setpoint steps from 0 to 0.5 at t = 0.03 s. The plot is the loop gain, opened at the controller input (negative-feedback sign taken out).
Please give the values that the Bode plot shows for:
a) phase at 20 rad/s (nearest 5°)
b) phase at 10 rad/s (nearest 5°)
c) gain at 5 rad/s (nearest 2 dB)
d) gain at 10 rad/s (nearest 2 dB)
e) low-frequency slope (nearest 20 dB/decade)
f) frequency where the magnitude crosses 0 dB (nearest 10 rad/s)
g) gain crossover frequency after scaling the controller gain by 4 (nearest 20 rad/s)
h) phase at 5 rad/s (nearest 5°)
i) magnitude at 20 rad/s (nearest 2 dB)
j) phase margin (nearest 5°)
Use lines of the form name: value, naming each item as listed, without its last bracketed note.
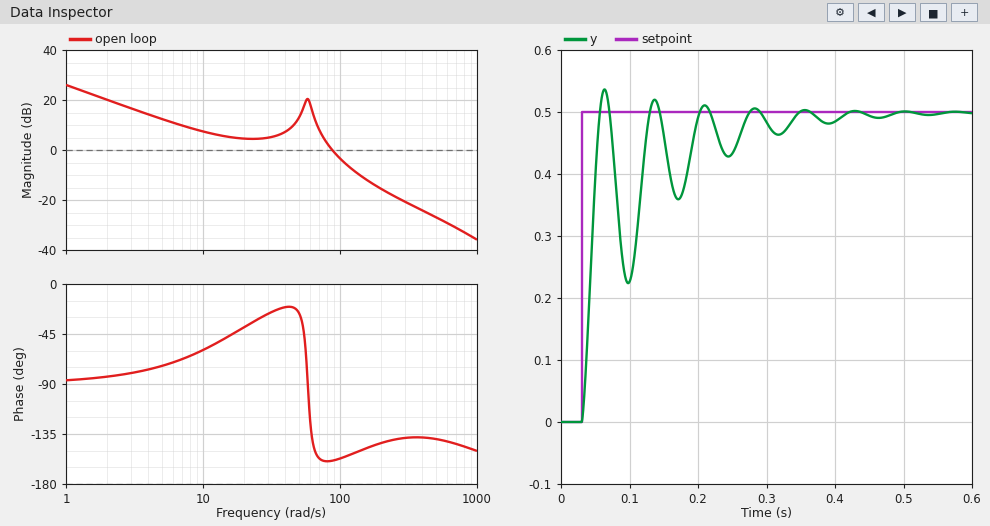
phase at 20 rad/s: -40°
phase at 10 rad/s: -60°
gain at 5 rad/s: 12 dB
gain at 10 rad/s: 8 dB
low-frequency slope: -20 dB/decade
frequency where the magnitude crosses 0 dB: 90 rad/s
gain crossover frequency after scaling the controller gain by 4: 160 rad/s
phase at 5 rad/s: -75°
magnitude at 20 rad/s: 4 dB
phase margin: 20°
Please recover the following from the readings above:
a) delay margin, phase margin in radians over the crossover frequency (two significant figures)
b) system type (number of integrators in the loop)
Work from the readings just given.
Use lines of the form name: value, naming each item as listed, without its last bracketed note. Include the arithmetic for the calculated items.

delay margin, phase margin in radians over the crossover frequency: 20 × π / 180 / 90 = 0.0039 s
system type: 1
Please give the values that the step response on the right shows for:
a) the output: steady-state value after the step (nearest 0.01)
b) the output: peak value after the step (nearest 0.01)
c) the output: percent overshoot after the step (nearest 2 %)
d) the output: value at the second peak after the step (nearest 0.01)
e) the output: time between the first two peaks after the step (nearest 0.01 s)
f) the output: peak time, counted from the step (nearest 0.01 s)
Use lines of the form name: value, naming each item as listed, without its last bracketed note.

the output: steady-state value after the step: 0.50
the output: peak value after the step: 0.54
the output: percent overshoot after the step: 8 %
the output: value at the second peak after the step: 0.52
the output: time between the first two peaks after the step: 0.07 s
the output: peak time, counted from the step: 0.03 s
